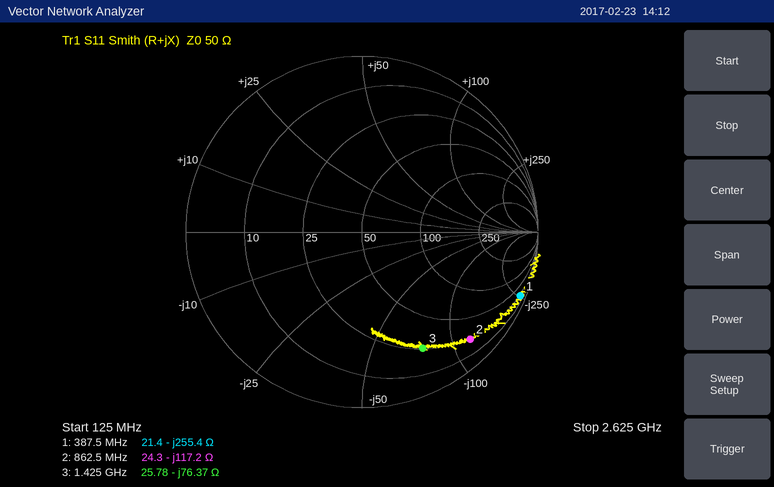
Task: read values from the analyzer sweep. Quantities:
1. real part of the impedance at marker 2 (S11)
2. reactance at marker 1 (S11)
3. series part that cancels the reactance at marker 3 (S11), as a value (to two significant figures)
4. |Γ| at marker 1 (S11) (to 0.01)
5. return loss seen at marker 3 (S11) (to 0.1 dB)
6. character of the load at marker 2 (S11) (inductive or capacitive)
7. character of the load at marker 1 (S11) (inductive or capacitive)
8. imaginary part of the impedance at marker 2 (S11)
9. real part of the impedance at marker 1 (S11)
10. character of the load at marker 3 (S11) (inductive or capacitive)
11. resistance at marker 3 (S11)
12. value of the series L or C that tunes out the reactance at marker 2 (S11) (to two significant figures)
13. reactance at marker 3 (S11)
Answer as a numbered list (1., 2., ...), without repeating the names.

1. 24.3 Ω
2. -255.4 Ω
3. 8.5 nH
4. 0.97
5. 2.6 dB
6. capacitive
7. capacitive
8. -117.2 Ω
9. 21.4 Ω
10. capacitive
11. 25.78 Ω
12. 22 nH
13. -76.37 Ω
